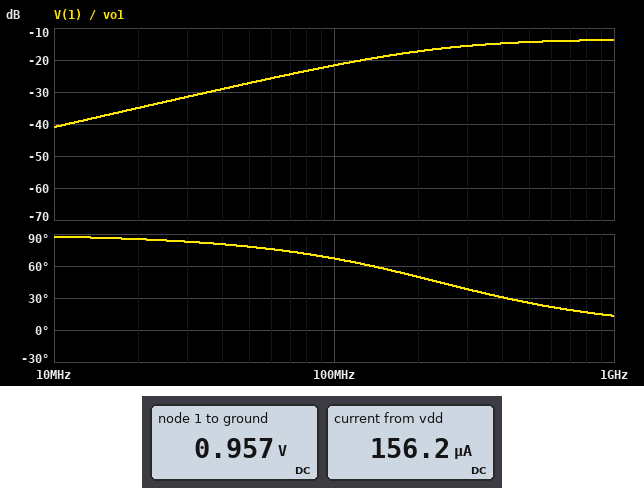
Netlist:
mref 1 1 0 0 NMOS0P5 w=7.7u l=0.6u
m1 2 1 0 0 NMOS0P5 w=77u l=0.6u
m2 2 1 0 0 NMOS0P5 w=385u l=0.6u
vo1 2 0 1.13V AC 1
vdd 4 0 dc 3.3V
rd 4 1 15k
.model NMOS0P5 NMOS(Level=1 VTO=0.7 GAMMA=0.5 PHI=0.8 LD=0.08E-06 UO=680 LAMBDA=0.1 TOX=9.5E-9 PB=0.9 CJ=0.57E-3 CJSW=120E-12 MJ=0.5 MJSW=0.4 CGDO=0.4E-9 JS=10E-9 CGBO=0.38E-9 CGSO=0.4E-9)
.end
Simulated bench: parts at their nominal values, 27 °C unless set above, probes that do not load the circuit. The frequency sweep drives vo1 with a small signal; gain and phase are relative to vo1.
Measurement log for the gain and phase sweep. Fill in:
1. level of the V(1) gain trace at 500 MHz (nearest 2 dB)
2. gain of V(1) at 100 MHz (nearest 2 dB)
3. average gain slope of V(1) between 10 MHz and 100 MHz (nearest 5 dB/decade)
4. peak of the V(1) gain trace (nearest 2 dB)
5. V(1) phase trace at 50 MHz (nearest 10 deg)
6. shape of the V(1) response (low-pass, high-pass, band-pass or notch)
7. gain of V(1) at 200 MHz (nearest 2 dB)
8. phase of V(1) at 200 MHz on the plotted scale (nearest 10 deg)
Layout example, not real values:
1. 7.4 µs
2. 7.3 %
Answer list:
1. -14 dB
2. -22 dB
3. 20 dB/decade
4. -14 dB
5. 80 deg
6. high-pass
7. -18 dB
8. 50 deg
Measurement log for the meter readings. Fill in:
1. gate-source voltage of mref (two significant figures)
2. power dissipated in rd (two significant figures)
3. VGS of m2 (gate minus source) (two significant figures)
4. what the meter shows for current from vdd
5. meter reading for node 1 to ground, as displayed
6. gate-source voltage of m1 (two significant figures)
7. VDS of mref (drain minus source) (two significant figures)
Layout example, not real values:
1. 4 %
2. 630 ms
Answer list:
1. 960 mV
2. 370 µW
3. 960 mV
4. 156.2 µA
5. 0.957 V
6. 960 mV
7. 960 mV
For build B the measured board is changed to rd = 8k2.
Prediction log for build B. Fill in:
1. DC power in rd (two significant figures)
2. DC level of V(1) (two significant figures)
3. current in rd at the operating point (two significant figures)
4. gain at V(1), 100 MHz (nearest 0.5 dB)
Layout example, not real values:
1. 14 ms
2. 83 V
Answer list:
1. 620 µW
2. 1.0 V
3. 280 µA
4. -24.0 dB
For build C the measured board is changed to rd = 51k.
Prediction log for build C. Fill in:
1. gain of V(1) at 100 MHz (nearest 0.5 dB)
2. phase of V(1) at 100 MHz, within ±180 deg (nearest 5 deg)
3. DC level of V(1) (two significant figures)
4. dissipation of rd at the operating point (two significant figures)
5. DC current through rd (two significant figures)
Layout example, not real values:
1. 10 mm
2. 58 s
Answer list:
1. -17.5 dB
2. 50 deg
3. 840 mV
4. 120 µW
5. 48 µA
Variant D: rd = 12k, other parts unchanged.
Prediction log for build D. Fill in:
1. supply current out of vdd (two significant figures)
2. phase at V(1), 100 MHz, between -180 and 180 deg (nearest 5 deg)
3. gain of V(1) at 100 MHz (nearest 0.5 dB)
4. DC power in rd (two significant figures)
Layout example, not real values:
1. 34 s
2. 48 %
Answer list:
1. 190 µA
2. 70 deg
3. -22.5 dB
4. 450 µW
